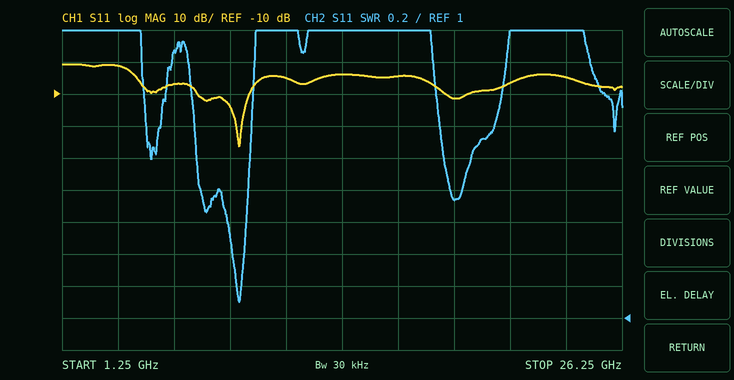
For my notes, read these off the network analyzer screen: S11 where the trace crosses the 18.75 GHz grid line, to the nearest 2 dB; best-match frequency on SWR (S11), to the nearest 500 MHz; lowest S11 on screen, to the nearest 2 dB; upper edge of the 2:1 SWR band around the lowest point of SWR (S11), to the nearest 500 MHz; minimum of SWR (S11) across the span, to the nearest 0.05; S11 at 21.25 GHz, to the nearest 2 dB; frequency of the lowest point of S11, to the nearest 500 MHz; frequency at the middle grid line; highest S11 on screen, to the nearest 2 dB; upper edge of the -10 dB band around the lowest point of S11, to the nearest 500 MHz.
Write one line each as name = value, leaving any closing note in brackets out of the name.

S11 where the trace crosses the 18.75 GHz grid line, to the nearest 2 dB = -12 dB
best-match frequency on SWR (S11), to the nearest 500 MHz = 9.0 GHz
lowest S11 on screen, to the nearest 2 dB = -26 dB
upper edge of the 2:1 SWR band around the lowest point of SWR (S11), to the nearest 500 MHz = 9.5 GHz
minimum of SWR (S11) across the span, to the nearest 0.05 = 1.10
S11 at 21.25 GHz, to the nearest 2 dB = -6 dB
frequency of the lowest point of S11, to the nearest 500 MHz = 9.0 GHz
frequency at the middle grid line = 13.75 GHz
highest S11 on screen, to the nearest 2 dB = 0 dB
upper edge of the -10 dB band around the lowest point of S11, to the nearest 500 MHz = 9.5 GHz
